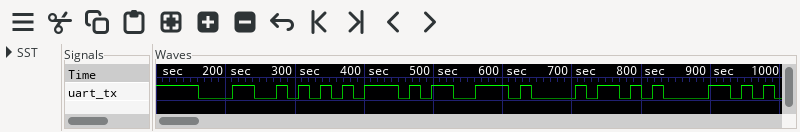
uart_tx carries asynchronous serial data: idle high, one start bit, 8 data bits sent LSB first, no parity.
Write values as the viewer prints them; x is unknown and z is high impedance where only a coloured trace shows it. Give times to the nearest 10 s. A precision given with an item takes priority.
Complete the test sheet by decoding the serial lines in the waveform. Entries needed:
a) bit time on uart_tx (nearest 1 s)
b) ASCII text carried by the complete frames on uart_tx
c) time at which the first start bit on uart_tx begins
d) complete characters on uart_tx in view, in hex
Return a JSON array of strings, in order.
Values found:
["16 s", "\"Lusha\"", "160 s", "4C, 75, 73, 68, 61"]
